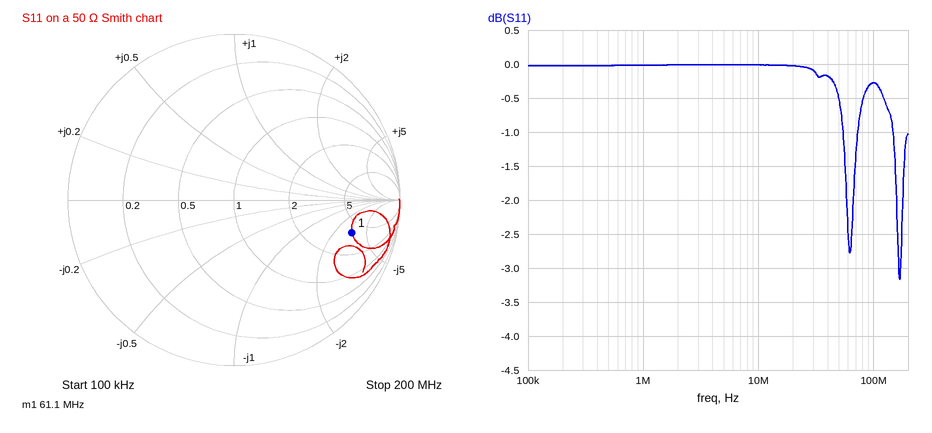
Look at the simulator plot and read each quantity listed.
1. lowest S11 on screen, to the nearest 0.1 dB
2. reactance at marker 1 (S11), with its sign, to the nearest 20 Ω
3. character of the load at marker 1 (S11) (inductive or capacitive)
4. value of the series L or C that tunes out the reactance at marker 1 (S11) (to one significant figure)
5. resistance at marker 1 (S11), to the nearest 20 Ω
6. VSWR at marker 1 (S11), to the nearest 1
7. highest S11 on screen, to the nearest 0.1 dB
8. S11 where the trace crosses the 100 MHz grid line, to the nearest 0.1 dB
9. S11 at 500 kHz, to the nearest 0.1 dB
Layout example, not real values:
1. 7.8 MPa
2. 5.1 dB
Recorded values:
1. -3.2 dB
2. -160 Ω
3. capacitive
4. 400 nH
5. 180 Ω
6. 7
7. 0.0 dB
8. -0.3 dB
9. 0.0 dB
